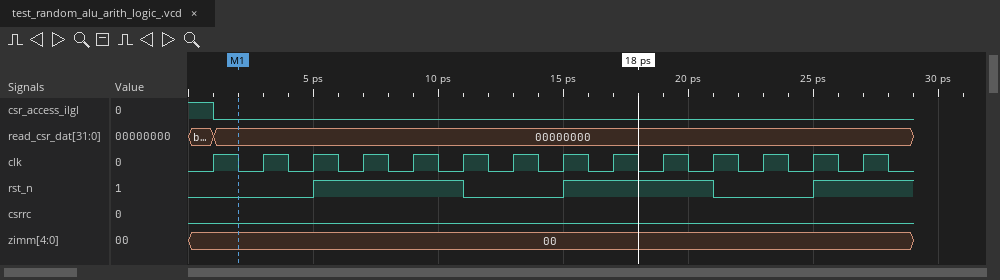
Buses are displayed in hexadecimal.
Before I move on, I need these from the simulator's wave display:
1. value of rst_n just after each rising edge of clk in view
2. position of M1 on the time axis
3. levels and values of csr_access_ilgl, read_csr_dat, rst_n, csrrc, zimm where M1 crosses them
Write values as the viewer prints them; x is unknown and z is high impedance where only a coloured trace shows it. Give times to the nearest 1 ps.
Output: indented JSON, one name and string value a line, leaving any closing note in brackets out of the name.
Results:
{
  "value of rst_n just after each rising edge of clk in view": "0 0 1 1 1 0 0 1 1 1 0 0 1 1",
  "position of M1 on the time axis": "2 ps",
  "levels and values of csr_access_ilgl, read_csr_dat, rst_n, csrrc, zimm where M1 crosses them": "csr_access_ilgl=0, read_csr_dat=00000000, rst_n=0, csrrc=0, zimm=00"
}
